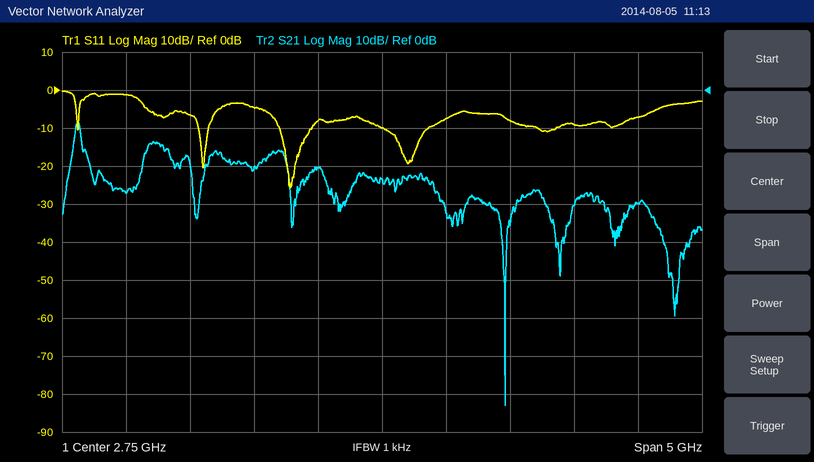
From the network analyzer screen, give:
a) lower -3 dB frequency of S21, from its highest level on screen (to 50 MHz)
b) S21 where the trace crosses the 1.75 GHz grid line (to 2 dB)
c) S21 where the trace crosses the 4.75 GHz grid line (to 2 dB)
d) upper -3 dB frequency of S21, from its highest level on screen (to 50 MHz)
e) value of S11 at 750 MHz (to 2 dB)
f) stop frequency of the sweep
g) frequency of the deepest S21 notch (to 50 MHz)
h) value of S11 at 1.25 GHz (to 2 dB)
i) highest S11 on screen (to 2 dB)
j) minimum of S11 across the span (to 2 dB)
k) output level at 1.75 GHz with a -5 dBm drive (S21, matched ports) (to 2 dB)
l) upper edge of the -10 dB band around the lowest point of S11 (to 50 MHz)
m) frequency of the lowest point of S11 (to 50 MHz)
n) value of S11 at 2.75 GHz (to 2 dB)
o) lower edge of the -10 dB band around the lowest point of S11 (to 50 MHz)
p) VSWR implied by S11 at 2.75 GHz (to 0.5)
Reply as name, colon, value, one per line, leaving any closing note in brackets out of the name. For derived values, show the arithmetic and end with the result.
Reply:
lower -3 dB frequency of S21, from its highest level on screen: 350 MHz
S21 where the trace crosses the 1.75 GHz grid line: -20 dB
S21 where the trace crosses the 4.75 GHz grid line: -30 dB
upper -3 dB frequency of S21, from its highest level on screen: 400 MHz
value of S11 at 750 MHz: -2 dB
stop frequency of the sweep: 5.25 GHz
frequency of the deepest S21 notch: 3.70 GHz
value of S11 at 1.25 GHz: -6 dB
highest S11 on screen: 0 dB
minimum of S11 across the span: -26 dB
output level at 1.75 GHz with a -5 dBm drive (S21, matched ports): -5 dBm + (-20 dB) = -26 dBm
upper edge of the -10 dB band around the lowest point of S11: 2.20 GHz
frequency of the lowest point of S11: 2.05 GHz
value of S11 at 2.75 GHz: -10 dB
lower edge of the -10 dB band around the lowest point of S11: 1.95 GHz
VSWR implied by S11 at 2.75 GHz: |Γ| = 10^(-10/20) = 0.3162; VSWR = (1 + 0.3162)/(1 − 0.3162) ≈ 1.92, so 2.0 to the nearest 0.5
